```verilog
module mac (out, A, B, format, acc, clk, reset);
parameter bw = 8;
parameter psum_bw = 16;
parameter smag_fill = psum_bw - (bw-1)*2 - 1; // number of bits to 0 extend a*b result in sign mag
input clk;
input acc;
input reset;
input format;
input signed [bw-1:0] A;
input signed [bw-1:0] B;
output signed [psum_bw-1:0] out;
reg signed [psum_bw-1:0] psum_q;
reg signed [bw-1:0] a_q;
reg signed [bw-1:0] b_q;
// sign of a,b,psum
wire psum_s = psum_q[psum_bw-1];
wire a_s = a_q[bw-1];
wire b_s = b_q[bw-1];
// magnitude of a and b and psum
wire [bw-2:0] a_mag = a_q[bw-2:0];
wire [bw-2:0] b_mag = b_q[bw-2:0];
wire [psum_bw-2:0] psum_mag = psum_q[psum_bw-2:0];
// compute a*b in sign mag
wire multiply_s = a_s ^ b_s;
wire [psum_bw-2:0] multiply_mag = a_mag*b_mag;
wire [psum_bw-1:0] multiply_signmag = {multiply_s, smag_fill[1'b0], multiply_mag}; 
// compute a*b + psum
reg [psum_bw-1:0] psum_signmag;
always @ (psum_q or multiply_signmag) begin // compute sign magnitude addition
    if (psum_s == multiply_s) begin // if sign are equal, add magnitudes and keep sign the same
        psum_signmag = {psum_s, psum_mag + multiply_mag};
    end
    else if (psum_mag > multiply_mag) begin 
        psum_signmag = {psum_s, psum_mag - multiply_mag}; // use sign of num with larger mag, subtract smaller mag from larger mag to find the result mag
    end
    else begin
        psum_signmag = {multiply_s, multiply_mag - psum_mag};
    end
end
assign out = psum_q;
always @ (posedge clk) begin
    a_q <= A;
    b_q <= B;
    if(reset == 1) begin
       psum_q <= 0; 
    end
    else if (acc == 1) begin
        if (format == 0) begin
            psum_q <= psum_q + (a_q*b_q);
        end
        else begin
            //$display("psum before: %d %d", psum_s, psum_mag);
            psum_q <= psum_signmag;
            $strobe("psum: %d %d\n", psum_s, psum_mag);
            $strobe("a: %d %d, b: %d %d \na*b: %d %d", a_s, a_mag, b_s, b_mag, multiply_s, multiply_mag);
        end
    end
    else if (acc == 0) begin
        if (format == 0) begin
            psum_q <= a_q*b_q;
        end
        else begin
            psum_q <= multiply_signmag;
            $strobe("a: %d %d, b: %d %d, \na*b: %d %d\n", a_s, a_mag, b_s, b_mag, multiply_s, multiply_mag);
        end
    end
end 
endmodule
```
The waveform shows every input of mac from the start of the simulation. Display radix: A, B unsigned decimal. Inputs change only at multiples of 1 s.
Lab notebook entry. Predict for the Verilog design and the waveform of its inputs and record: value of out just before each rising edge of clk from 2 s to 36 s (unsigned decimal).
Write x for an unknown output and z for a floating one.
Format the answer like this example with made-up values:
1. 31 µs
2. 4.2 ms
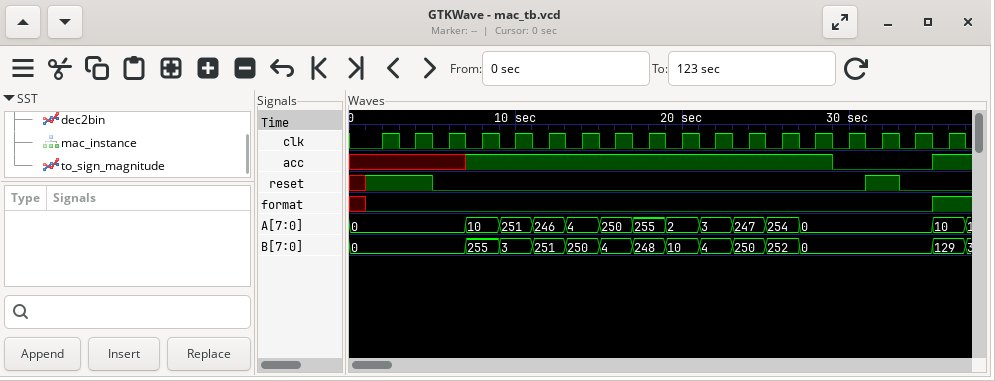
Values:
1. x, 0, 0, 0, 0, 65526, 65511, 25, 1, 65513, 65521, 5, 17, 71, 79, 0, 0, 0
